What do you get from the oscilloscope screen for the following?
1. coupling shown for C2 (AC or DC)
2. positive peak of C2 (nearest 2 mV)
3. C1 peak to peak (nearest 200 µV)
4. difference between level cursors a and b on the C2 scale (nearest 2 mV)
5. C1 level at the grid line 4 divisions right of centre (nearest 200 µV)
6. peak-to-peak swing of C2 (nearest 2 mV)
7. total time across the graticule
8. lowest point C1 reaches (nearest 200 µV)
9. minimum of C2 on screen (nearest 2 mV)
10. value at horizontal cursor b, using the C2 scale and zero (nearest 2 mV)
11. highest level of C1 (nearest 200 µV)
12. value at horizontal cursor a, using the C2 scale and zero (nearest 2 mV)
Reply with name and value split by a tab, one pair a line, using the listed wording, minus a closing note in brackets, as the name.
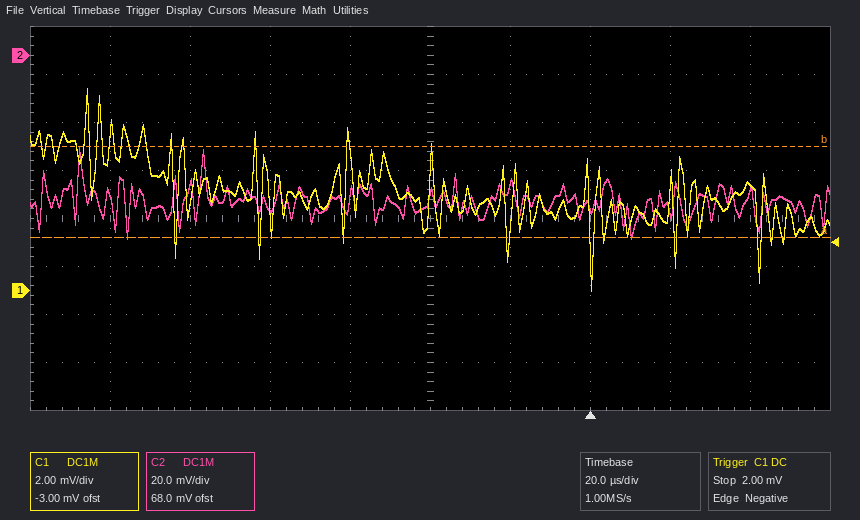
coupling shown for C2	DC
positive peak of C2	-38 mV
C1 peak to peak	8.4 mV
difference between level cursors a and b on the C2 scale	38 mV
C1 level at the grid line 4 divisions right of centre	4.4 mV
peak-to-peak swing of C2	38 mV
total time across the graticule	200 µs
lowest point C1 reaches	0.0 mV
minimum of C2 on screen	-76 mV
value at horizontal cursor b, using the C2 scale and zero	-38 mV
highest level of C1	8.4 mV
value at horizontal cursor a, using the C2 scale and zero	-76 mV
